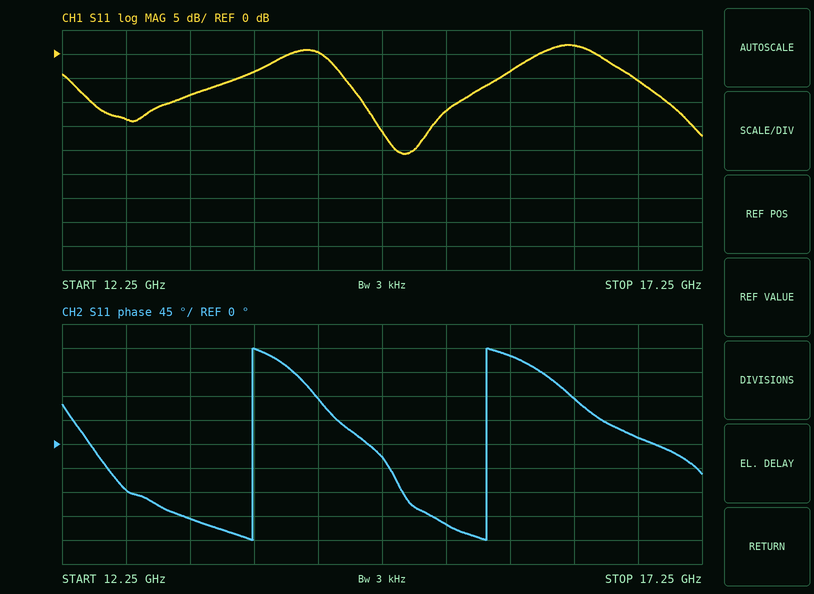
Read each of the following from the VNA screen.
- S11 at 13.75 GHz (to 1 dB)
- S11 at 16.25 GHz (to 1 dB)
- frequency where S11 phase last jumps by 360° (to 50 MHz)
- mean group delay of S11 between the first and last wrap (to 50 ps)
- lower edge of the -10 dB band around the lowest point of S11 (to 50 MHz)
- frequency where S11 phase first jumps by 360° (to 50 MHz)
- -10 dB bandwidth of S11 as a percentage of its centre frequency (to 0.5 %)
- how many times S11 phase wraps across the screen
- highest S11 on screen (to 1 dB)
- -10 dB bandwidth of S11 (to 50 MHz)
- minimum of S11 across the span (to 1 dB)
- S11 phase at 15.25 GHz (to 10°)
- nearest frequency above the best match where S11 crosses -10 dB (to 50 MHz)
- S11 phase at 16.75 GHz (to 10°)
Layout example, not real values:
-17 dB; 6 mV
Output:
-4 dB; 2 dB; 15.55 GHz; 550 ps; 14.60 GHz; 13.75 GHz; 5.0 %; 2; 2 dB; 750 MHz; -21 dB; -150°; 15.35 GHz; 10°
